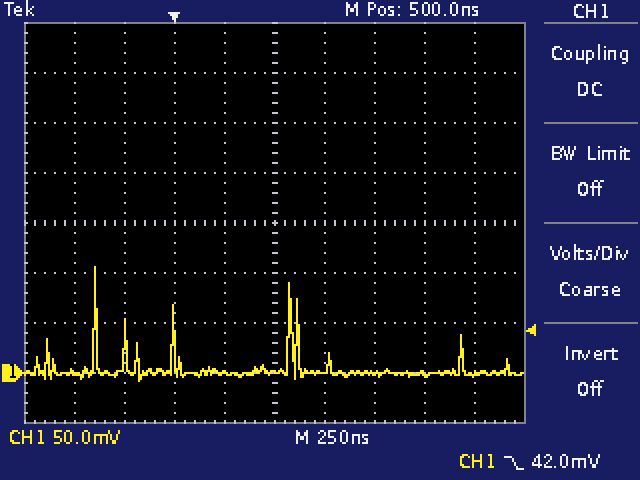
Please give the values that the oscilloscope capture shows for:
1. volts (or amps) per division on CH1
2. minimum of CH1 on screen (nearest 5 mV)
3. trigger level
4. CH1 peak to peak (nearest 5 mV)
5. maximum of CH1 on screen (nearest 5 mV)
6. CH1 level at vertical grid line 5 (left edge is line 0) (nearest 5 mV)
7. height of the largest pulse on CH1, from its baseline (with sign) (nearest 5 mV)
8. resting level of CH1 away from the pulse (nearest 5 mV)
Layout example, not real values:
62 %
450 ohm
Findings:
50 mV
-10 mV
42.0 mV
115 mV
105 mV
0 mV
+105 mV
0 mV
